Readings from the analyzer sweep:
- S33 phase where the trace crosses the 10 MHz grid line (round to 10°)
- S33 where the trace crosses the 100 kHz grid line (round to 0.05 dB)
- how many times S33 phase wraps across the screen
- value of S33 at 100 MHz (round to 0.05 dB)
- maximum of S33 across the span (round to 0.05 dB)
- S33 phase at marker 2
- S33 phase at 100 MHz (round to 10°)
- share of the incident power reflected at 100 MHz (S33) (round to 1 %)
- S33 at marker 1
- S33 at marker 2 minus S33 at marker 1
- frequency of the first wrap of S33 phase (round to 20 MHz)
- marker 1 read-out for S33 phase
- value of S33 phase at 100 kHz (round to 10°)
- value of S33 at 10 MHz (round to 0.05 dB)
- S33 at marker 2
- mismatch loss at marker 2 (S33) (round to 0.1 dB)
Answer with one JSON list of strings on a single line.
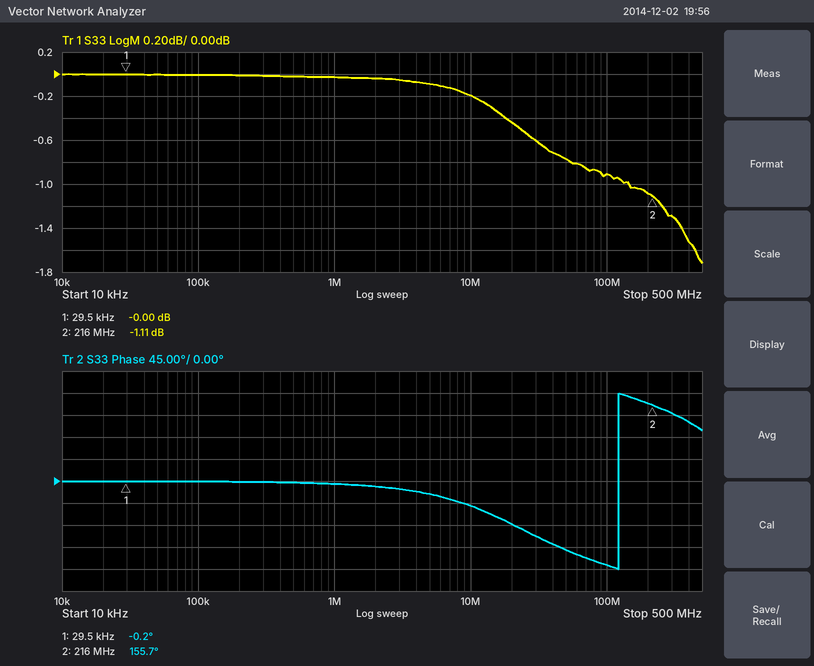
["-50°", "0.00 dB", "1", "-0.90 dB", "0.00 dB", "155.7°", "-170°", "81 %", "-0.00 dB", "-1.11 dB", "120 MHz", "-0.2°", "0°", "-0.20 dB", "-1.11 dB", "6.5 dB"]
